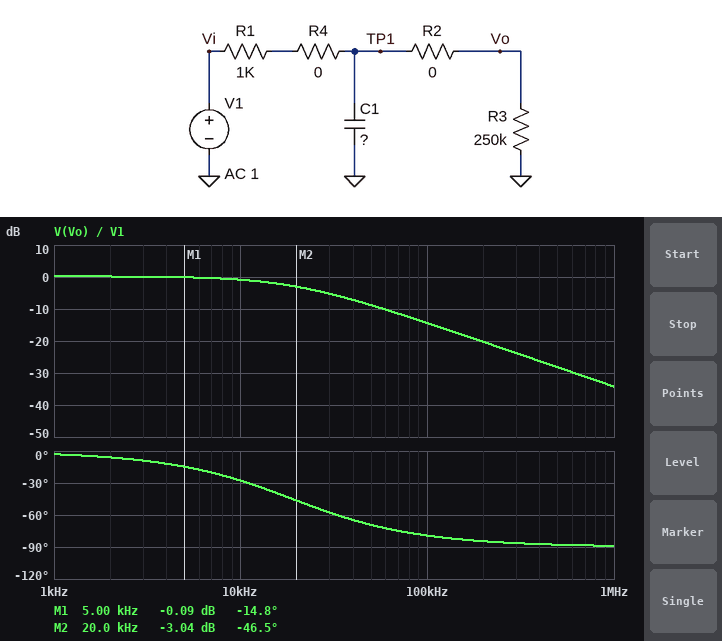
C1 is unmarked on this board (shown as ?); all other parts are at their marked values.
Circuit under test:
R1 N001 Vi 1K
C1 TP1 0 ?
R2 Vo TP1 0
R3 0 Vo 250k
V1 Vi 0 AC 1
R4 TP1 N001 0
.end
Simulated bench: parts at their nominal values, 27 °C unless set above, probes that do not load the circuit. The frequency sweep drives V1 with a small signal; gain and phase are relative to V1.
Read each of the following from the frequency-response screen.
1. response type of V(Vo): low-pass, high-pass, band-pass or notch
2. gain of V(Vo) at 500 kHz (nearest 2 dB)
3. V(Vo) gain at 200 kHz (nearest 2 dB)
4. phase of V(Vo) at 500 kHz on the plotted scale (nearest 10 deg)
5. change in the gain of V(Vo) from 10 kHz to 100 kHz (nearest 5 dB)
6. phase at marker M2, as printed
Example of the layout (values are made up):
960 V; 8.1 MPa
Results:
low-pass; -28 dB; -20 dB; -90 deg; -15 dB; -46.5 deg
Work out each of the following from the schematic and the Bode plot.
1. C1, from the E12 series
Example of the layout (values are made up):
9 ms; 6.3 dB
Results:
8.2 nF
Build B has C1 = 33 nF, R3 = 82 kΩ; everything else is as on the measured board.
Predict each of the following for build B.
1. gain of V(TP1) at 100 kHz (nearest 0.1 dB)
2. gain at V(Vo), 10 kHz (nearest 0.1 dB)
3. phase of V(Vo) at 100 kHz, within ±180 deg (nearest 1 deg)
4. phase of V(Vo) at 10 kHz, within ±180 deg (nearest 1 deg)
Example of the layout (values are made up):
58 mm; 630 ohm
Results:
-26.3 dB; -7.2 dB; -87 deg; -65 deg
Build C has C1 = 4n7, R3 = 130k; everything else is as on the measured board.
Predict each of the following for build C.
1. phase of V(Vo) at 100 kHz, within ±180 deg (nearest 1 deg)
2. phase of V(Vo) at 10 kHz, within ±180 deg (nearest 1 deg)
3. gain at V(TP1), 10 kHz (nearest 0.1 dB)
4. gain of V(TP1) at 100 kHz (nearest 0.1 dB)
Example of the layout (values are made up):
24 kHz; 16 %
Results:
-72 deg; -17 deg; -0.2 dB; -9.9 dB
